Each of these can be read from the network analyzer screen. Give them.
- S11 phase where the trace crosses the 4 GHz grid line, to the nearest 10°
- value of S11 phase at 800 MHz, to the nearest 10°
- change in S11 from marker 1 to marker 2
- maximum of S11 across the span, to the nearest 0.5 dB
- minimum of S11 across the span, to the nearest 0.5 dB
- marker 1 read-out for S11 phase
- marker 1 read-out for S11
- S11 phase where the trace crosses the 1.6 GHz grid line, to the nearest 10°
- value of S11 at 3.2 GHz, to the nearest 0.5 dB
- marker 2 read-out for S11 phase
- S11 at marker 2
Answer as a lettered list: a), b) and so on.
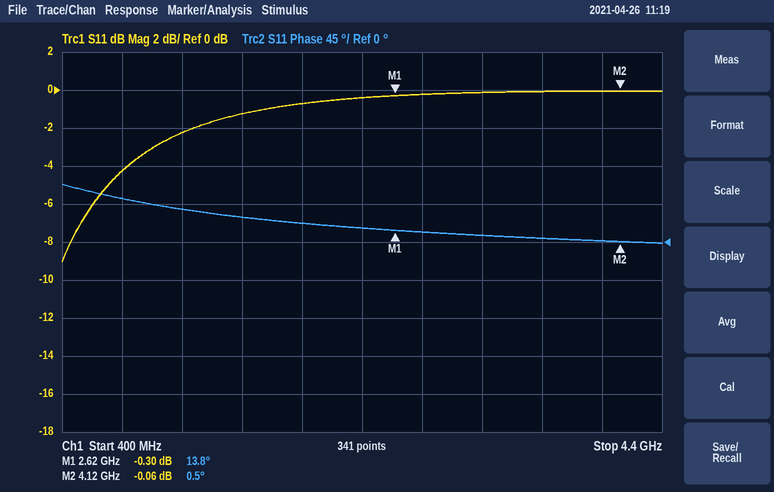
a) 0°
b) 50°
c) 0.24 dB
d) 0.0 dB
e) -9.0 dB
f) 13.8°
g) -0.30 dB
h) 30°
i) 0.0 dB
j) 0.5°
k) -0.06 dB
